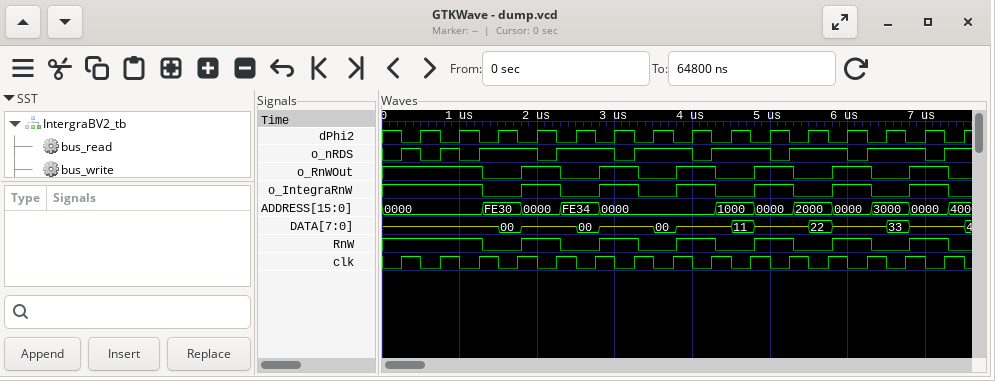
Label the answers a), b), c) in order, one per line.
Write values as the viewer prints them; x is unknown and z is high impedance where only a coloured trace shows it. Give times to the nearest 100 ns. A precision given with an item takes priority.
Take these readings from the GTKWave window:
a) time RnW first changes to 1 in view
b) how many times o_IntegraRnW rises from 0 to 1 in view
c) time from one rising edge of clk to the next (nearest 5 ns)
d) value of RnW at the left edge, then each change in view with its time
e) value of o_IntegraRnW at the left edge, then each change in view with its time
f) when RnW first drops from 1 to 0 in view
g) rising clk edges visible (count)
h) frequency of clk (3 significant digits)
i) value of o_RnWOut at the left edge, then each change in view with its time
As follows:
a) 1800 ns
b) 6
c) 500 ns
d) 1, 0 at 1300 ns, 1 at 1800 ns, 0 at 2300 ns, 1 at 2800 ns, 0 at 3300 ns, 1 at 3800 ns, 0 at 4300 ns, 1 at 4800 ns, 0 at 5300 ns, 1 at 5800 ns, 0 at 6300 ns, 1 at 6800 ns, 0 at 7300 ns
e) 1, 0 at 1300 ns, 1 at 1800 ns, 0 at 2300 ns, 1 at 2800 ns, 0 at 3300 ns, 1 at 3800 ns, 0 at 4300 ns, 1 at 4800 ns, 0 at 5300 ns, 1 at 5800 ns, 0 at 6300 ns, 1 at 6800 ns, 0 at 7300 ns
f) 1300 ns
g) 15
h) 2.00 MHz
i) 1, 0 at 1300 ns, 1 at 1800 ns, 0 at 2300 ns, 1 at 2800 ns, 0 at 3300 ns, 1 at 3800 ns, 0 at 4300 ns, 1 at 4800 ns, 0 at 5300 ns, 1 at 5800 ns, 0 at 6300 ns, 1 at 6800 ns, 0 at 7300 ns
